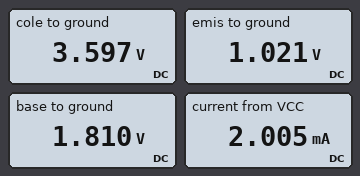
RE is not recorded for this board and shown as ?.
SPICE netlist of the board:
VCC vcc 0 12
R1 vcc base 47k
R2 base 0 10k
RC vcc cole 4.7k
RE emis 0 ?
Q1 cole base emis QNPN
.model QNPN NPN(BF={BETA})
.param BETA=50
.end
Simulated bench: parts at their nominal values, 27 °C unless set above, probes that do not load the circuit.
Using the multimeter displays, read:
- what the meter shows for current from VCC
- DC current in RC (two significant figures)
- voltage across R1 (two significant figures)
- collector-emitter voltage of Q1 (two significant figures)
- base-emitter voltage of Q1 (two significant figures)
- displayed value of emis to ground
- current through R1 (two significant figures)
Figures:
2.005 mA
1.8 mA
10 V
2.6 V
790 mV
1.021 V
220 µA
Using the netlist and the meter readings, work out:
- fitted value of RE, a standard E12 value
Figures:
560 Ω
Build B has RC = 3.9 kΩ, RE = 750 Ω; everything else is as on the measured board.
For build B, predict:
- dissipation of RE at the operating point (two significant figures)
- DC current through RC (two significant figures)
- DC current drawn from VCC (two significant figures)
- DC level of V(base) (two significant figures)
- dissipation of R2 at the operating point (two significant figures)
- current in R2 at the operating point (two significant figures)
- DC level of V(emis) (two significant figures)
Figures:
1.6 mW
1.4 mA
1.6 mA
1.9 V
350 µW
190 µA
1.1 V
